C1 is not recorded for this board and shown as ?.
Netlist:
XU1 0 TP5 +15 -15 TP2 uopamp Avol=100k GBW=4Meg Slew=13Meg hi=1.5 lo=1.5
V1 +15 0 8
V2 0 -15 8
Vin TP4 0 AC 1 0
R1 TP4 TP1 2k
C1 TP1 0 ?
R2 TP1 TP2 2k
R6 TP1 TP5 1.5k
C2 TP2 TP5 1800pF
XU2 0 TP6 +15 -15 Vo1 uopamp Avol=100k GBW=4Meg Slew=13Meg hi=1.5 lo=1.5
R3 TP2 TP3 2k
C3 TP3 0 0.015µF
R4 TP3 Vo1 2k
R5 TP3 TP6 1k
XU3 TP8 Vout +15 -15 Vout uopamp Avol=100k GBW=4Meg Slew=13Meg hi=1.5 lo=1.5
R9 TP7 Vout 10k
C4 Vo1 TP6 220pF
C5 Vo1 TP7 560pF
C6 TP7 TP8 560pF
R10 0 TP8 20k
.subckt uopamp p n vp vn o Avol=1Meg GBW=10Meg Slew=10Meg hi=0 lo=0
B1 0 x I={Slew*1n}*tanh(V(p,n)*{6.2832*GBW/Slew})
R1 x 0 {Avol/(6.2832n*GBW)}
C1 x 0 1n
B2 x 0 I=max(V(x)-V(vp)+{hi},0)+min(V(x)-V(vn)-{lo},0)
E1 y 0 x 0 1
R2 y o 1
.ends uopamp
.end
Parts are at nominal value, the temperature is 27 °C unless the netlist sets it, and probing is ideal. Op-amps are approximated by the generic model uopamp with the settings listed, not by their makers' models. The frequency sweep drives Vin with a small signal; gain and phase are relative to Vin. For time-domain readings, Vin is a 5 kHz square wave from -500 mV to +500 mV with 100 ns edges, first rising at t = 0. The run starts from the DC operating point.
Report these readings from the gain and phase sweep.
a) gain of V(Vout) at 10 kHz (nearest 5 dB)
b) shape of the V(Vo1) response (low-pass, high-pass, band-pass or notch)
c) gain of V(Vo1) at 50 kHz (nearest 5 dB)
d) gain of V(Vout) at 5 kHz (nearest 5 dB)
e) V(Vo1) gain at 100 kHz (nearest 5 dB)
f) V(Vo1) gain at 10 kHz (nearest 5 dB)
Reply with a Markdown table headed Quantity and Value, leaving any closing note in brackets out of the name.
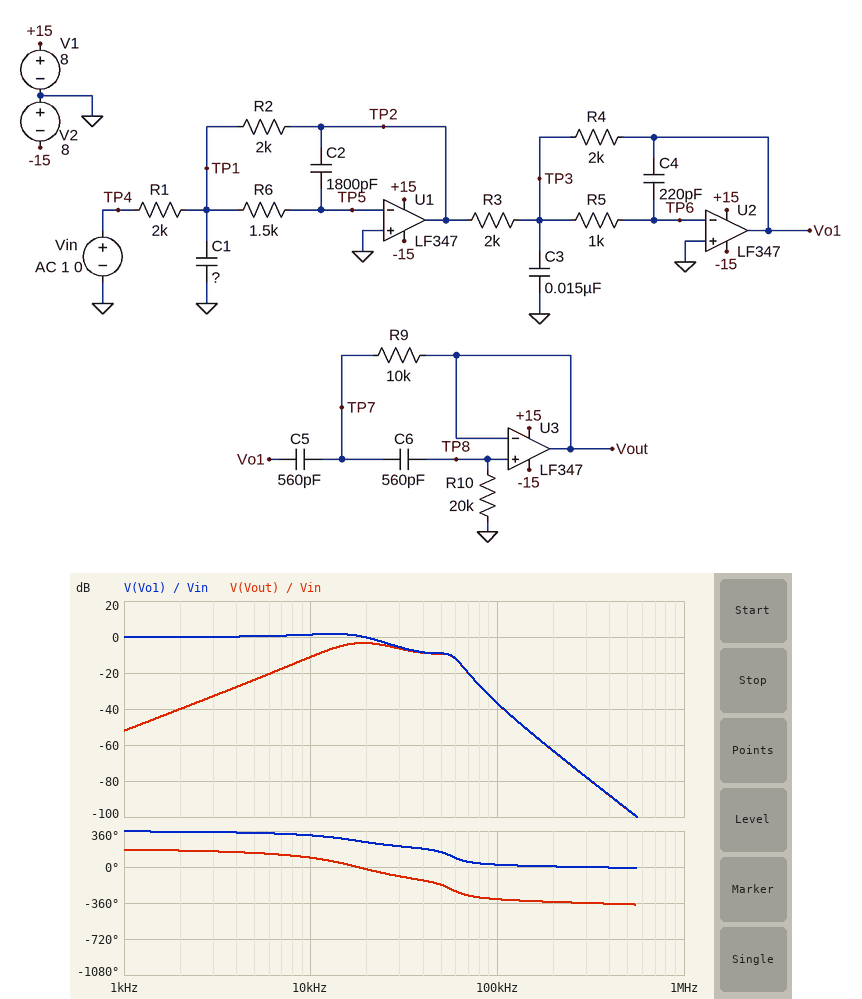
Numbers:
| Quantity | Value |
|---|---|
| gain of V(Vout) at 10 kHz | -10 dB |
| shape of the V(Vo1) response | low-pass |
| gain of V(Vo1) at 50 kHz | -10 dB |
| gain of V(Vout) at 5 kHz | -25 dB |
| V(Vo1) gain at 100 kHz | -35 dB |
| V(Vo1) gain at 10 kHz | 0 dB |
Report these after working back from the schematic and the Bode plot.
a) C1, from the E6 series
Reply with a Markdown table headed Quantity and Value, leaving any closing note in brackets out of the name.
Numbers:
| Quantity | Value |
|---|---|
| C1, from the E6 series | 15 nF |
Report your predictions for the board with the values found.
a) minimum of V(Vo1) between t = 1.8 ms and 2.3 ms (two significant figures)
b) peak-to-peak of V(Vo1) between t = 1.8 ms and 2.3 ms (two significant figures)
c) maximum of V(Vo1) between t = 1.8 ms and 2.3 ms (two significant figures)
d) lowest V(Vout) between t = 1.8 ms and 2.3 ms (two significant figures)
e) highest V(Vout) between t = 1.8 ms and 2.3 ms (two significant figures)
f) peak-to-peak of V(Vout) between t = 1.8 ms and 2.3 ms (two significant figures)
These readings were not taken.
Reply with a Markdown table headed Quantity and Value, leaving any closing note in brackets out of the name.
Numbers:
| Quantity | Value |
|---|---|
| minimum of V(Vo1) between t = 1.8 ms and 2.3 ms | -690 mV |
| peak-to-peak of V(Vo1) between t = 1.8 ms and 2.3 ms | 1.4 V |
| maximum of V(Vo1) between t = 1.8 ms and 2.3 ms | 690 mV |
| lowest V(Vout) between t = 1.8 ms and 2.3 ms | -280 mV |
| highest V(Vout) between t = 1.8 ms and 2.3 ms | 280 mV |
| peak-to-peak of V(Vout) between t = 1.8 ms and 2.3 ms | 560 mV |
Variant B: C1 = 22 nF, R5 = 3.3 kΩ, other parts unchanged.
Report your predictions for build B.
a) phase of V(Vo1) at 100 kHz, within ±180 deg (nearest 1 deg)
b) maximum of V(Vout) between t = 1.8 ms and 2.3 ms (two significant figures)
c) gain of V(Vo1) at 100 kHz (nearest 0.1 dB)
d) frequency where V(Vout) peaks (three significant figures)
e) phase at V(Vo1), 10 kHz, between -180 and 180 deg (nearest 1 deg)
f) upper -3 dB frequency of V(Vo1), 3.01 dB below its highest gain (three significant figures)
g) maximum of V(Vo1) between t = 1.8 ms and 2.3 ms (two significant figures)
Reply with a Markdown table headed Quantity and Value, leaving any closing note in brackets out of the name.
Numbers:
| Quantity | Value |
|---|---|
| phase of V(Vo1) at 100 kHz, within ±180 deg | 13 deg |
| maximum of V(Vout) between t = 1.8 ms and 2.3 ms | 250 mV |
| gain of V(Vo1) at 100 kHz | -51.7 dB |
| frequency where V(Vout) peaks | 17.3 kHz |
| phase at V(Vo1), 10 kHz, between -180 and 180 deg | -55 deg |
| upper -3 dB frequency of V(Vo1), 3.01 dB below its highest gain | 19.1 kHz |
| maximum of V(Vo1) between t = 1.8 ms and 2.3 ms | 830 mV |
